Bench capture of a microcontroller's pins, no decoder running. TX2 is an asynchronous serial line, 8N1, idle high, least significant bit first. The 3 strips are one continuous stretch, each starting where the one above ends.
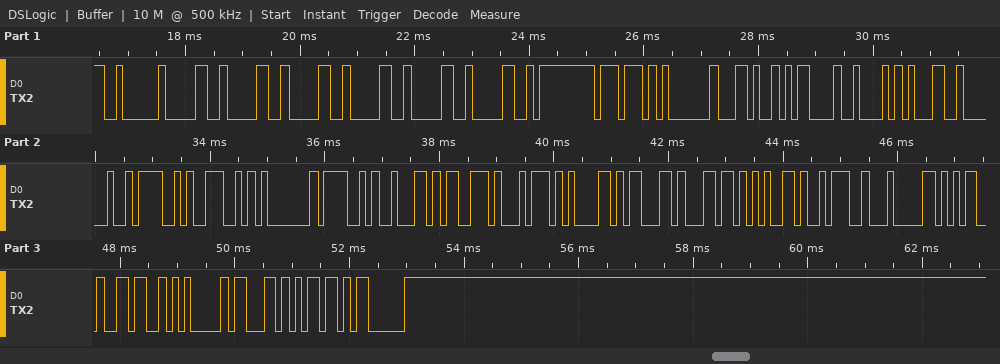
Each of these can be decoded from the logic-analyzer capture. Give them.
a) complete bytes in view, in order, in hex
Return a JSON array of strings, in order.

["02 30 30 30 30 30 30 FF 77 01 2C 0D 42 31 20 4F 4E 01 4F 62 73 74 61 63 6C 65 3A 04 35 36 05 63 6D 03"]
